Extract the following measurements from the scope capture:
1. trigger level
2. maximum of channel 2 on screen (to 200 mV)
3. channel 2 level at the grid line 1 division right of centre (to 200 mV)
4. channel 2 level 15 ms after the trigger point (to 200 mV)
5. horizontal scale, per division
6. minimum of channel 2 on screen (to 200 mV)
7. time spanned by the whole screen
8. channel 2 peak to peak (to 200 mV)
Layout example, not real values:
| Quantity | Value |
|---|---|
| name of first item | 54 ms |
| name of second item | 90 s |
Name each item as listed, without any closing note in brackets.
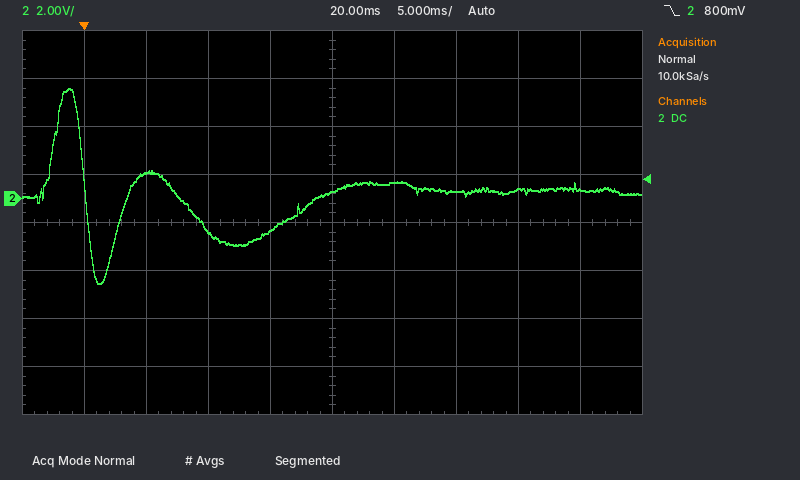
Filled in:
| Quantity | Value |
|---|---|
| trigger level | 800 mV |
| maximum of channel 2 on screen | 4.6 V |
| channel 2 level at the grid line 1 division right of centre | 600 mV |
| channel 2 level 15 ms after the trigger point | -1.4 V |
| horizontal scale, per division | 5 ms |
| minimum of channel 2 on screen | -3.6 V |
| time spanned by the whole screen | 50 ms |
| channel 2 peak to peak | 8.2 V |
